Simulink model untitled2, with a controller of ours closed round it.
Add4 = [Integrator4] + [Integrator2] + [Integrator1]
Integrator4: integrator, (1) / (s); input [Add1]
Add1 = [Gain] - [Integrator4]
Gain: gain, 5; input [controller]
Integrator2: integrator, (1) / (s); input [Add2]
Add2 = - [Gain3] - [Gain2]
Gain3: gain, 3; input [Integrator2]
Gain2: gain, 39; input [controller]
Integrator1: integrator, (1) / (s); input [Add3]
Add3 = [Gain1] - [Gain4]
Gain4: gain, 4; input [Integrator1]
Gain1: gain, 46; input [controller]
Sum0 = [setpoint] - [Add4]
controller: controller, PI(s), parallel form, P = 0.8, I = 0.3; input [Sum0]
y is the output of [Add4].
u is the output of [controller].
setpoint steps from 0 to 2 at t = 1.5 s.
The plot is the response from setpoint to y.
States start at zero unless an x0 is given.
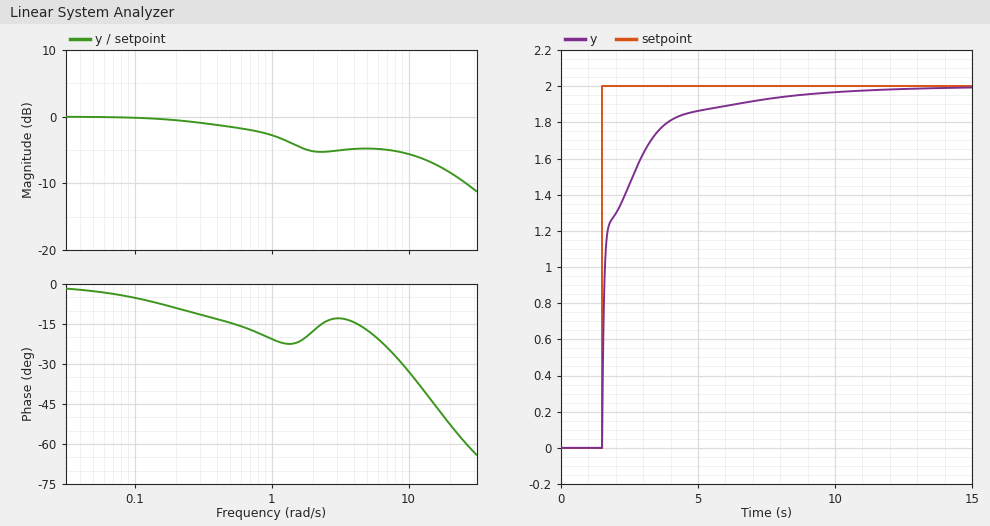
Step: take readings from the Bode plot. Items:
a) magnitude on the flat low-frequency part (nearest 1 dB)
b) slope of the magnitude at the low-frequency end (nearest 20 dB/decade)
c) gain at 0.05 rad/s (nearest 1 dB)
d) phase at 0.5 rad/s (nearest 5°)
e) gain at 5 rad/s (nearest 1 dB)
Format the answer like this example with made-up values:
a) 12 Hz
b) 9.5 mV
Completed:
a) 0 dB
b) 0 dB/decade
c) 0 dB
d) -15°
e) -5 dB
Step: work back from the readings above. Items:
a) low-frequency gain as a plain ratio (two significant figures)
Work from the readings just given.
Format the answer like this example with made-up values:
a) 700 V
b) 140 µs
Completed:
a) 1.0
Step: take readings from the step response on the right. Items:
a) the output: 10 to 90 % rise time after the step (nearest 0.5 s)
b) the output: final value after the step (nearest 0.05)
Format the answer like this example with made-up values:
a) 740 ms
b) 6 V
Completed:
a) 2.5 s
b) 2.00
